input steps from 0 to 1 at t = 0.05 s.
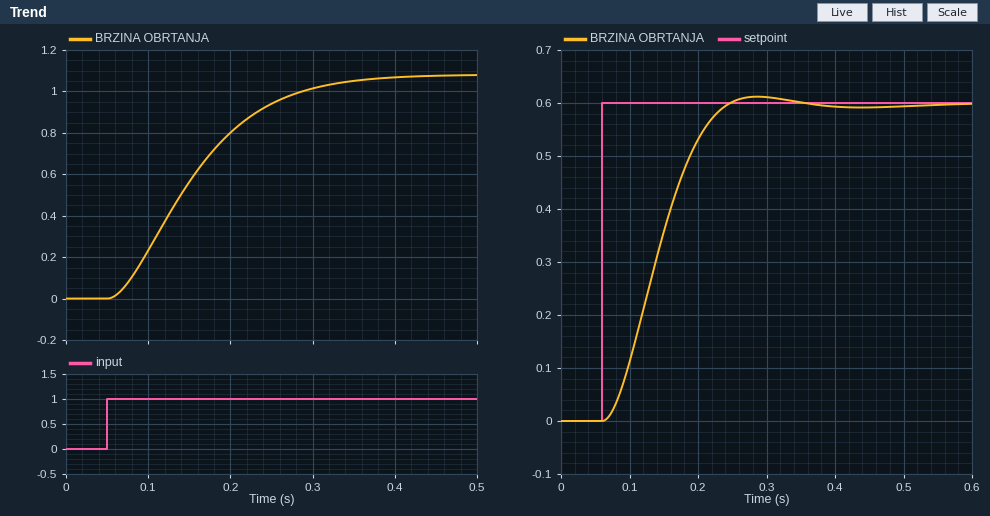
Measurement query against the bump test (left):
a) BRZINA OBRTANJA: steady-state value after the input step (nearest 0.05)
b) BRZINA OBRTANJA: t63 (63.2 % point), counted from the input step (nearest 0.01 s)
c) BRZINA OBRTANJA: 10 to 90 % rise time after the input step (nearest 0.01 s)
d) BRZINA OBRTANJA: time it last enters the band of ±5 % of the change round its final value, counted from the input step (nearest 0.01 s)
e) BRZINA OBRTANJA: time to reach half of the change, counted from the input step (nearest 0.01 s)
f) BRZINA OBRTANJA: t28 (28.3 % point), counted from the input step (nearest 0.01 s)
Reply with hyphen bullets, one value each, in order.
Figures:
- 1.10
- 0.12 s
- 0.19 s
- 0.26 s
- 0.10 s
- 0.06 s
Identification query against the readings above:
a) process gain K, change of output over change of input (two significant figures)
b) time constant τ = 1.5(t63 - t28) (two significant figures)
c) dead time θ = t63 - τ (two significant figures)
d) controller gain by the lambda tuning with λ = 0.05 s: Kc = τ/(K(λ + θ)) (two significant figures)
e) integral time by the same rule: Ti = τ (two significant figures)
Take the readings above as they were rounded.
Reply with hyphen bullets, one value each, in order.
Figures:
- 1.1
- 0.090 s
- 0.030 s
- 1.0
- 0.090 s
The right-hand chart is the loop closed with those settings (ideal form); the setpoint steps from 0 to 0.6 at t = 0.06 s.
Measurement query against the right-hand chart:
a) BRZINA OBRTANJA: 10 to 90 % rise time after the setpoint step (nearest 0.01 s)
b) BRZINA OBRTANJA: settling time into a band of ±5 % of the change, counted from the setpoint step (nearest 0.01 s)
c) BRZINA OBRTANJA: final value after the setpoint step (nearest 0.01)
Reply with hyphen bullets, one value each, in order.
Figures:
- 0.12 s
- 0.16 s
- 0.60
